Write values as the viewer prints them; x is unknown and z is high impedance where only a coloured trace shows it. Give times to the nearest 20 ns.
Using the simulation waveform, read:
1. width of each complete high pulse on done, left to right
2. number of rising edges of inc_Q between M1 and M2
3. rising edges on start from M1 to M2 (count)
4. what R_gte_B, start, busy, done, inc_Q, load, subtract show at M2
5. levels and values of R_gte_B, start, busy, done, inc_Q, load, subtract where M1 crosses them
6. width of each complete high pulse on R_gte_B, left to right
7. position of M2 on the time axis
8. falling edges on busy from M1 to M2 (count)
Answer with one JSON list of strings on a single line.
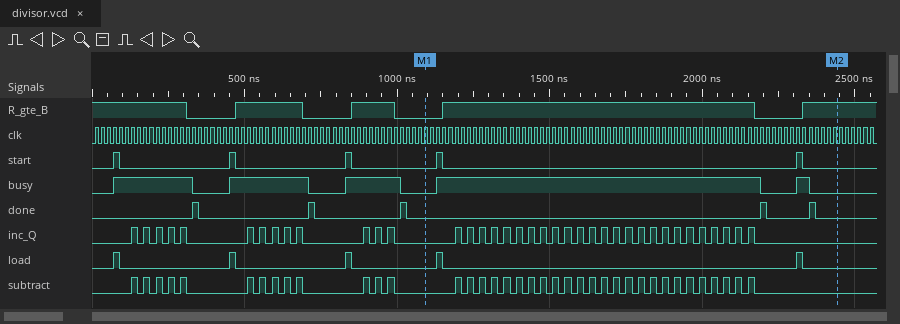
["20 ns, 20 ns, 20 ns, 20 ns, 20 ns", "25", "2", "R_gte_B=1, start=0, busy=0, done=0, inc_Q=0, load=0, subtract=0", "R_gte_B=0, start=0, busy=0, done=0, inc_Q=0, load=0, subtract=0", "220 ns, 140 ns, 1020 ns", "2440 ns", "2"]
